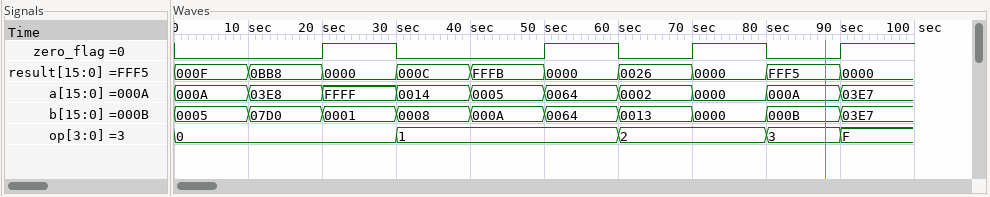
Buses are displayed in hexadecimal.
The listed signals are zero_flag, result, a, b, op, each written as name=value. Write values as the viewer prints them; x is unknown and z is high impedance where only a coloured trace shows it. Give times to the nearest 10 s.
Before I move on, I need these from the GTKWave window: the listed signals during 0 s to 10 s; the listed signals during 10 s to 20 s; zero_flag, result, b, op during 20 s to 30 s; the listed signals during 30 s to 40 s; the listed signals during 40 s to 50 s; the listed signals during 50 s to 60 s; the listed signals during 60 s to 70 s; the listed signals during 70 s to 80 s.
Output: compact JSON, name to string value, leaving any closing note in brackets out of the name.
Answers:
{"the listed signals during 0 s to 10 s": "zero_flag=0, result=000F, a=000A, b=0005, op=0", "the listed signals during 10 s to 20 s": "zero_flag=0, result=0BB8, a=03E8, b=07D0, op=0", "zero_flag, result, b, op during 20 s to 30 s": "zero_flag=1, result=0000, b=0001, op=0", "the listed signals during 30 s to 40 s": "zero_flag=0, result=000C, a=0014, b=0008, op=1", "the listed signals during 40 s to 50 s": "zero_flag=0, result=FFFB, a=0005, b=000A, op=1", "the listed signals during 50 s to 60 s": "zero_flag=1, result=0000, a=0064, b=0064, op=1", "the listed signals during 60 s to 70 s": "zero_flag=0, result=0026, a=0002, b=0013, op=2", "the listed signals during 70 s to 80 s": "zero_flag=1, result=0000, a=0000, b=0000, op=2"}
